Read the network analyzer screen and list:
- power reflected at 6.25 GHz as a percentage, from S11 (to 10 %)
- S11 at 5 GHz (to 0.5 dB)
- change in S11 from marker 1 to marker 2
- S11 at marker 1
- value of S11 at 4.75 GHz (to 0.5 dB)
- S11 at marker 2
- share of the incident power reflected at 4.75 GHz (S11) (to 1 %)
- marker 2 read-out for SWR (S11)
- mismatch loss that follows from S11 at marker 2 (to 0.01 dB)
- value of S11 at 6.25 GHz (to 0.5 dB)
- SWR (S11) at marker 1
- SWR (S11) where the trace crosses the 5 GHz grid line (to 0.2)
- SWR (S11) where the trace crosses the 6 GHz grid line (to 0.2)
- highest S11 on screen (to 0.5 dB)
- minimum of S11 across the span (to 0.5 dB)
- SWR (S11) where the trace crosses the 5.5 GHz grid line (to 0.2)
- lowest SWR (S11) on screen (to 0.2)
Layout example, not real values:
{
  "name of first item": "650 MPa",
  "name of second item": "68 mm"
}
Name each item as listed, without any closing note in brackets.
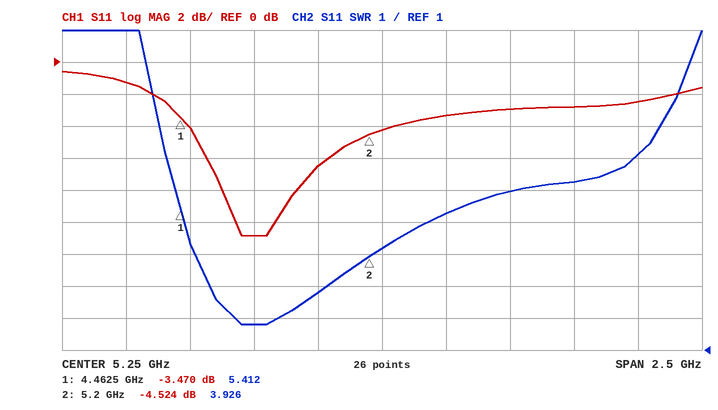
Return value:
{
  "power reflected at 6.25 GHz as a percentage, from S11": "60 %",
  "S11 at 5 GHz": "-6.5 dB",
  "change in S11 from marker 1 to marker 2": "-1.054 dB",
  "S11 at marker 1": "-3.470 dB",
  "value of S11 at 4.75 GHz": "-11.0 dB",
  "S11 at marker 2": "-4.524 dB",
  "share of the incident power reflected at 4.75 GHz (S11)": "8 %",
  "marker 2 read-out for SWR": "3.926",
  "mismatch loss that follows from S11 at marker 2": "1.89 dB",
  "value of S11 at 6.25 GHz": "-2.5 dB",
  "SWR (S11) at marker 1": "5.412",
  "SWR (S11) where the trace crosses the 5 GHz grid line": "2.8",
  "SWR (S11) where the trace crosses the 6 GHz grid line": "6.2",
  "highest S11 on screen": "-0.5 dB",
  "minimum of S11 across the span": "-11.0 dB",
  "SWR (S11) where the trace crosses the 5.5 GHz grid line": "5.2",
  "lowest SWR (S11) on screen": "1.8"
}
